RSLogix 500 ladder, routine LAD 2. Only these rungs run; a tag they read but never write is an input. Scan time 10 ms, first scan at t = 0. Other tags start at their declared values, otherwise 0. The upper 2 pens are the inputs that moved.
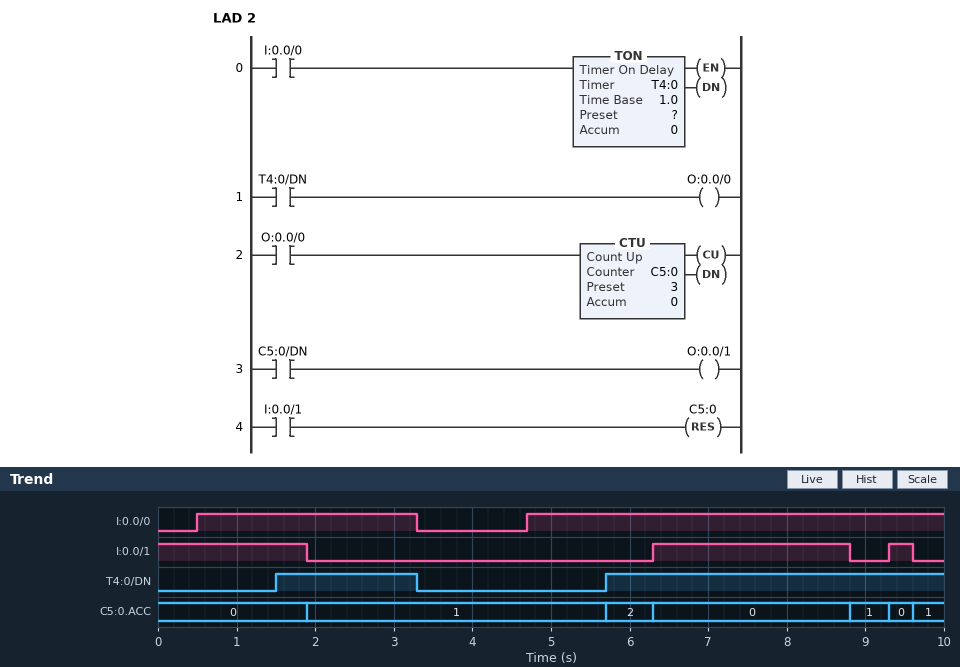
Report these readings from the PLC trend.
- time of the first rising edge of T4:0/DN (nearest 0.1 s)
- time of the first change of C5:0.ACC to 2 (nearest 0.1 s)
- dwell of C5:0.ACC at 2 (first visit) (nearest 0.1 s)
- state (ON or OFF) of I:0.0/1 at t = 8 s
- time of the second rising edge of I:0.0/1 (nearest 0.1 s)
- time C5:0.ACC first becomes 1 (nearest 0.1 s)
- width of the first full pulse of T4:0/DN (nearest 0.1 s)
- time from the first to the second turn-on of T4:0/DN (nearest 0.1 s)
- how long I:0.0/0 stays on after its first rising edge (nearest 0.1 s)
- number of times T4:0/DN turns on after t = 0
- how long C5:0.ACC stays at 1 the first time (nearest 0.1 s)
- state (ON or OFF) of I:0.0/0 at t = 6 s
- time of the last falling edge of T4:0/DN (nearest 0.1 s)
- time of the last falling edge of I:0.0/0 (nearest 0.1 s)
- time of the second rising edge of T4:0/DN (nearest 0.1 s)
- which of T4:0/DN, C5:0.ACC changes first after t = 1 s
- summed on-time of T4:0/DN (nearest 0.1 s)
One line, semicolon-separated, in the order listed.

1.5 s; 5.7 s; 0.6 s; ON; 9.3 s; 1.9 s; 1.8 s; 4.2 s; 2.8 s; 2; 3.8 s; ON; 3.3 s; 3.3 s; 5.7 s; T4:0/DN; 6.1 s
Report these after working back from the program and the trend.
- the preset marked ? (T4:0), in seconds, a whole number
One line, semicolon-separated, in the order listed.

1 s
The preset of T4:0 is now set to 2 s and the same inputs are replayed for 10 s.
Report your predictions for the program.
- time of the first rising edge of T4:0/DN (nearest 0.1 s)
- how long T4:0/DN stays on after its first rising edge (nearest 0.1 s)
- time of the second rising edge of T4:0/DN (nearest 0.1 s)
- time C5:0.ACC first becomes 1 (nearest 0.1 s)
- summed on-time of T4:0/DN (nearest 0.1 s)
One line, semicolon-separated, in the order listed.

2.5 s; 0.8 s; 6.7 s; 2.5 s; 4.1 s
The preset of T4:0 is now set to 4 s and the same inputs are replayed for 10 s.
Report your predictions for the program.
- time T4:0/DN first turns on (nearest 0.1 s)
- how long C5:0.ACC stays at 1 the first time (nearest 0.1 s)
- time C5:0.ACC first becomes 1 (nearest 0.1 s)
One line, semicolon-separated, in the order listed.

8.7 s; 0.5 s; 8.8 s
